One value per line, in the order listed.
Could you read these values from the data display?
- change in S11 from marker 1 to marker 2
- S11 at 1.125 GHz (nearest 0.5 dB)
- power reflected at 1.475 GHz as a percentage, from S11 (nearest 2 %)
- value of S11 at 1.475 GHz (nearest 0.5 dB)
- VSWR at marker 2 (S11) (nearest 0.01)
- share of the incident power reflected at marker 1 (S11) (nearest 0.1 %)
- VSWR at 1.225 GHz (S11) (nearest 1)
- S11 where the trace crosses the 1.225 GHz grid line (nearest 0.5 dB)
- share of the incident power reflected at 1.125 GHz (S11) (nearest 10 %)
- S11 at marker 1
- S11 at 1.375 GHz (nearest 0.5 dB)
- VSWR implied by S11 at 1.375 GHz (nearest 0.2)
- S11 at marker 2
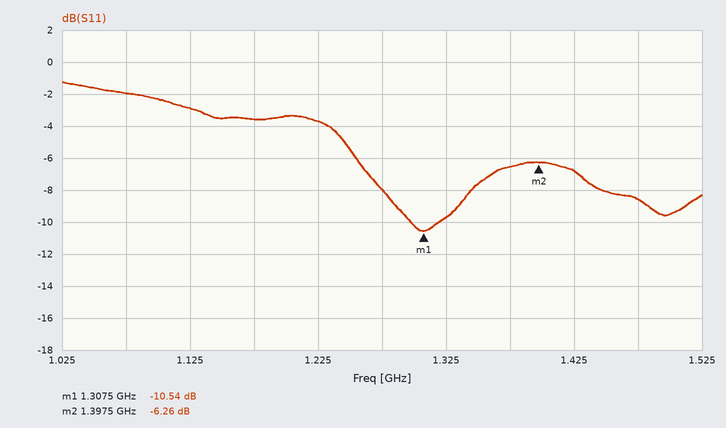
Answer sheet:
4.28 dB
-3.0 dB
14 %
-8.5 dB
2.89
8.8 %
5
-3.5 dB
50 %
-10.54 dB
-6.5 dB
2.8
-6.26 dB
